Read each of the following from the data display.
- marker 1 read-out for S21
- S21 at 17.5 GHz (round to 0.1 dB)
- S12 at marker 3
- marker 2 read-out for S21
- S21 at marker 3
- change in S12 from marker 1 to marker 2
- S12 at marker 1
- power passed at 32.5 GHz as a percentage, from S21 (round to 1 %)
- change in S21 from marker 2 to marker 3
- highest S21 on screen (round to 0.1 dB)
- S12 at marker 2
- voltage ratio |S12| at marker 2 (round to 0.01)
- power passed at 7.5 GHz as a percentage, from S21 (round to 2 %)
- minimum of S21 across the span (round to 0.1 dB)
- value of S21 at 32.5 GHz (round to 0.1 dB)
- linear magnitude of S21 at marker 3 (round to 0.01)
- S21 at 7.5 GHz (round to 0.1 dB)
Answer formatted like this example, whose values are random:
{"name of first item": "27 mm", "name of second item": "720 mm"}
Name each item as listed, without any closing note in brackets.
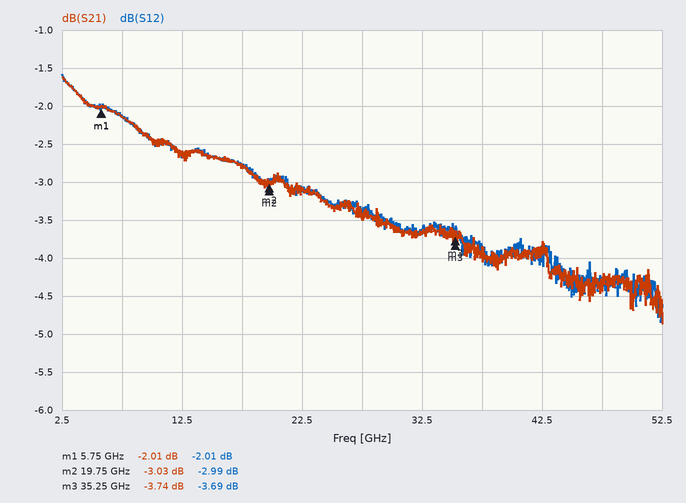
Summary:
{"marker 1 read-out for S21": "-2.01 dB", "S21 at 17.5 GHz": "-2.8 dB", "S12 at marker 3": "-3.69 dB", "marker 2 read-out for S21": "-3.03 dB", "S21 at marker 3": "-3.74 dB", "change in S12 from marker 1 to marker 2": "-0.98 dB", "S12 at marker 1": "-2.01 dB", "power passed at 32.5 GHz as a percentage, from S21": "43 %", "change in S21 from marker 2 to marker 3": "-0.71 dB", "highest S21 on screen": "-1.6 dB", "S12 at marker 2": "-2.99 dB", "voltage ratio |S12| at marker 2": "0.71", "power passed at 7.5 GHz as a percentage, from S21": "62 %", "minimum of S21 across the span": "-4.9 dB", "value of S21 at 32.5 GHz": "-3.7 dB", "linear magnitude of S21 at marker 3": "0.65", "S21 at 7.5 GHz": "-2.1 dB"}
